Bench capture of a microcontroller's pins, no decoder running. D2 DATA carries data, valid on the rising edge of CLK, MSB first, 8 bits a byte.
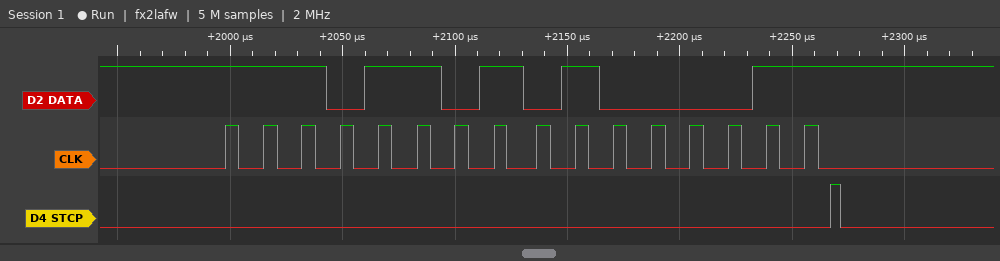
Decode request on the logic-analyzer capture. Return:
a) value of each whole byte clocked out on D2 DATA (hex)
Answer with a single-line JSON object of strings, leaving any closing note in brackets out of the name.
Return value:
{"value of each whole byte clocked out on D2 DATA": "0xED 0x43"}
